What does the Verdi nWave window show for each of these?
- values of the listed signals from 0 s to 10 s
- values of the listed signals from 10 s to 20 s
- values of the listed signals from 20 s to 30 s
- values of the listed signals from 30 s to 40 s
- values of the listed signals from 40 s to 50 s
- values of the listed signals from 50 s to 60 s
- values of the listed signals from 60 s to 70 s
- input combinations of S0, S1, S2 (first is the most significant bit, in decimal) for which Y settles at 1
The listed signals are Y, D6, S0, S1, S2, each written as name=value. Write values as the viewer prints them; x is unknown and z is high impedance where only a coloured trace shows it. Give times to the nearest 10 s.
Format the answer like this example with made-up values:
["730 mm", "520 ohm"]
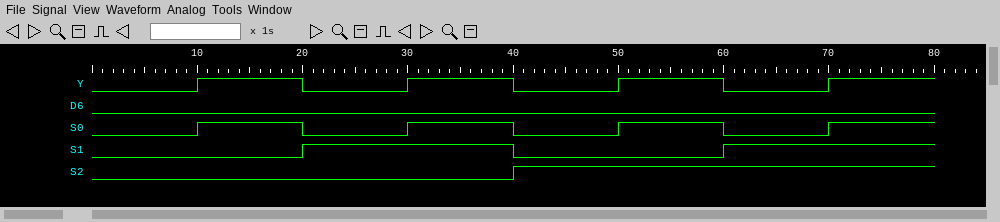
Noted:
["Y=0, D6=0, S0=0, S1=0, S2=0", "Y=1, D6=0, S0=1, S1=0, S2=0", "Y=0, D6=0, S0=0, S1=1, S2=0", "Y=1, D6=0, S0=1, S1=1, S2=0", "Y=0, D6=0, S0=0, S1=0, S2=1", "Y=1, D6=0, S0=1, S1=0, S2=1", "Y=0, D6=0, S0=0, S1=1, S2=1", "4, 5, 6, 7"]
